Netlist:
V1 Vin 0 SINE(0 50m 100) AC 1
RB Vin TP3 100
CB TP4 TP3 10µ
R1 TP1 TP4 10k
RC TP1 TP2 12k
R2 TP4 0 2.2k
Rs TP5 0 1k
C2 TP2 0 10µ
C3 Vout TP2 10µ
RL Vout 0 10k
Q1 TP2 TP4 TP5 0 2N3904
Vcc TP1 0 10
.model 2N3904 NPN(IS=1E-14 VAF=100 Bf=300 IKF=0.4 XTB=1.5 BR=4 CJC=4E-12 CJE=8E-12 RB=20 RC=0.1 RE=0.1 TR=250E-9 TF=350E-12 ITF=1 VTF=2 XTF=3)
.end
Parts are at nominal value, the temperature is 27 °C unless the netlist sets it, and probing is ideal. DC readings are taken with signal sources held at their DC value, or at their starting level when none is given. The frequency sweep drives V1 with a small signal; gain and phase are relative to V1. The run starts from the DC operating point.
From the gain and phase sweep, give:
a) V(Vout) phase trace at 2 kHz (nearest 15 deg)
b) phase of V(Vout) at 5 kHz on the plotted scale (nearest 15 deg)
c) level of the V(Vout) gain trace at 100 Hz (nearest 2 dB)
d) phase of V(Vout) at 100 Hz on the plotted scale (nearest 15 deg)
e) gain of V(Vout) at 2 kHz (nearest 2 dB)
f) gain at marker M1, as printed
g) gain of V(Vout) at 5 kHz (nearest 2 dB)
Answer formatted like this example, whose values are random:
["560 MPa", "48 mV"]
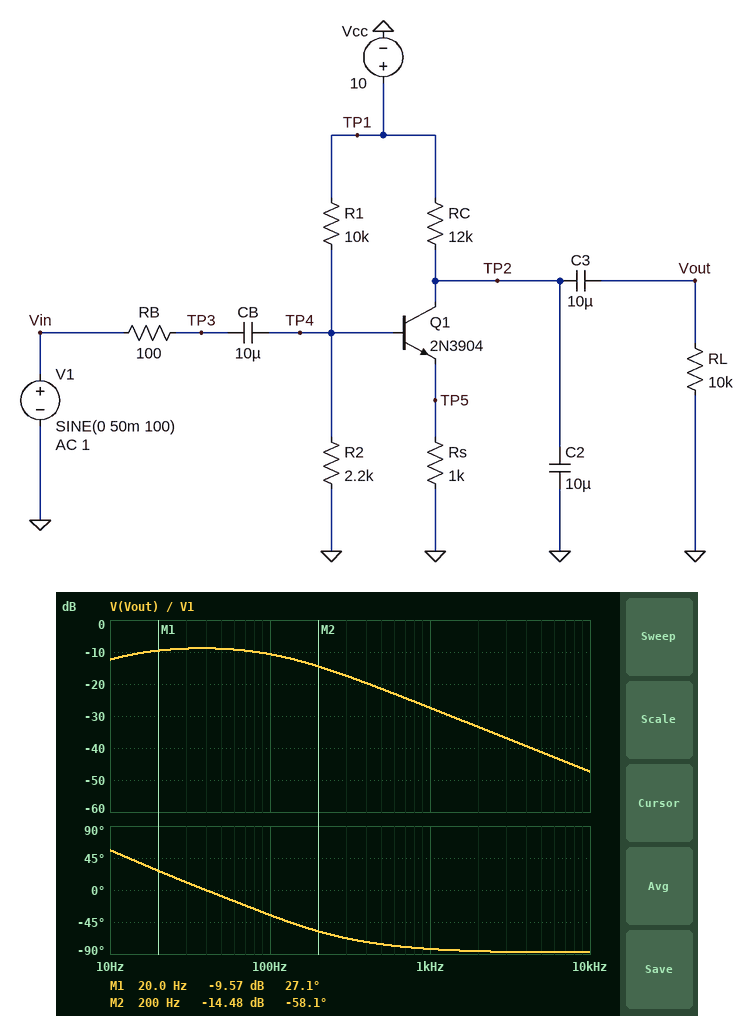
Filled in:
["-90 deg", "-90 deg", "-10 dB", "-30 deg", "-34 dB", "-9.57 dB", "-42 dB"]
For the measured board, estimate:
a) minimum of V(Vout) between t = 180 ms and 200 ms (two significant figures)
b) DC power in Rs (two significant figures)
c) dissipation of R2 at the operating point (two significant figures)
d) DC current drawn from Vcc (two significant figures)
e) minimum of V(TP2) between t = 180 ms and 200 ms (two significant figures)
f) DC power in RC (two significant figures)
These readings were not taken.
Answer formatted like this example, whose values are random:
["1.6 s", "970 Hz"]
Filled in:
["-13 mV", "800 µW", "1.1 mW", "1.6 mA", "910 mV", "6.9 mW"]
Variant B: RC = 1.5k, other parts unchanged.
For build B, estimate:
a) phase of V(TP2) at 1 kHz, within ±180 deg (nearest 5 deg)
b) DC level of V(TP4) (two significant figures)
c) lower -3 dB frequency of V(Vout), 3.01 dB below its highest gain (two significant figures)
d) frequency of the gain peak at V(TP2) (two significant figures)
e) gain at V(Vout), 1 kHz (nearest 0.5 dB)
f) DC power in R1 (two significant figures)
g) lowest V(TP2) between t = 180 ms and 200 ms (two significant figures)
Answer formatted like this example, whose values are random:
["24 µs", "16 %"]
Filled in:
["90 deg", "1.8 V", "4.4 Hz", "10 Hz", "-36.5 dB", "6.7 mW", "8.3 V"]
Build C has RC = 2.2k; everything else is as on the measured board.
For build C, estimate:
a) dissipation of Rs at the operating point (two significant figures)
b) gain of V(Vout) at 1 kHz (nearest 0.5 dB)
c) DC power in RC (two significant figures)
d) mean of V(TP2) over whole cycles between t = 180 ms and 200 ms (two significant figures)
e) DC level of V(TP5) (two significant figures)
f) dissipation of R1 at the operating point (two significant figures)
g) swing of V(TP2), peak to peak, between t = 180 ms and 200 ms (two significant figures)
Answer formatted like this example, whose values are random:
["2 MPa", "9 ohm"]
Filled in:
["1.3 mW", "-36.5 dB", "2.8 mW", "7.5 V", "1.1 V", "6.7 mW", "15 mV"]
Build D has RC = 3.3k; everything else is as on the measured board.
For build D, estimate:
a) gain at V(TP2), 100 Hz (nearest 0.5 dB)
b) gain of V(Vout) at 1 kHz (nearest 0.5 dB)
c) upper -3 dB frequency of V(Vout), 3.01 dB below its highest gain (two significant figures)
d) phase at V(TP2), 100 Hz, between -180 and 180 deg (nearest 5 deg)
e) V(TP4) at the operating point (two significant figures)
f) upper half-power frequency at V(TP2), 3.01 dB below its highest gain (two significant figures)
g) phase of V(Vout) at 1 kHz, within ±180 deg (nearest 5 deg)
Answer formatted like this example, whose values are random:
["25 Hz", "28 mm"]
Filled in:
["-16.5 dB", "-36.5 dB", "19 Hz", "100 deg", "1.8 V", "18 Hz", "90 deg"]
